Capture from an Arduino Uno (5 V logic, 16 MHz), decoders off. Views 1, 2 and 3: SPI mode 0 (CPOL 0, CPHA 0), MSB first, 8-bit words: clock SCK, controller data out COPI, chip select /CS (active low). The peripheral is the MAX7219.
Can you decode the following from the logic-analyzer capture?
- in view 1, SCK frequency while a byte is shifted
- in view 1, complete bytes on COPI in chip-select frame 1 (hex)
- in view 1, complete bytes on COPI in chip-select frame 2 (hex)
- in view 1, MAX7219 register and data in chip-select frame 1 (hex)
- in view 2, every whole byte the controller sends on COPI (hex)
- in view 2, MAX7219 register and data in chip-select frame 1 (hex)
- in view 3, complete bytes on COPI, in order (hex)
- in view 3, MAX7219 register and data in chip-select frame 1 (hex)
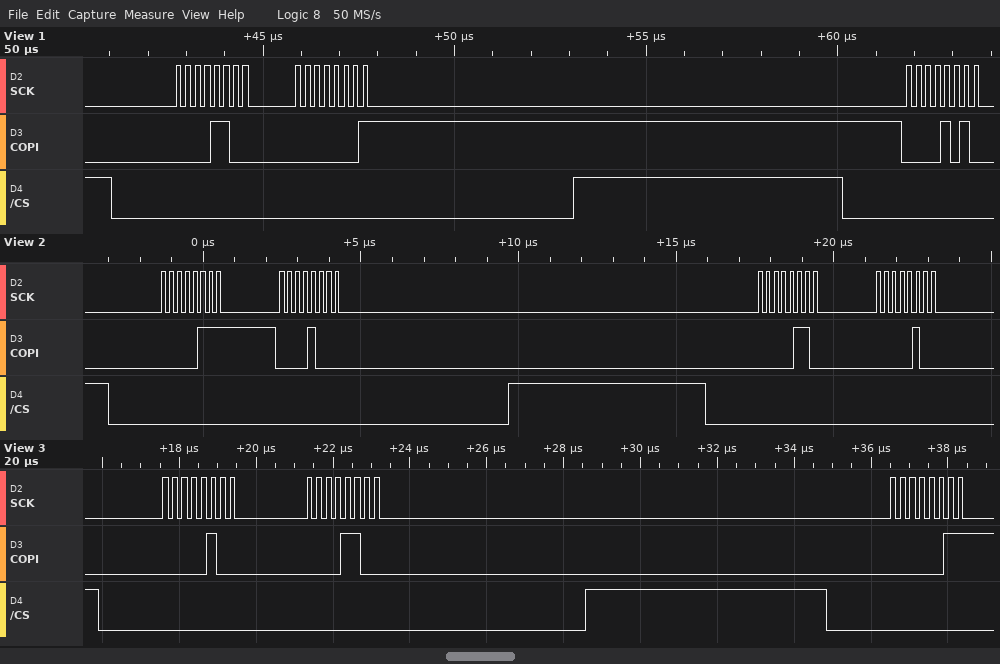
4 MHz
0C 01
0A
register 0xC, data 0x01
07 08 06 04
register 0x7, data 0x08
04 0C 03
register 0x4, data 0x0C
